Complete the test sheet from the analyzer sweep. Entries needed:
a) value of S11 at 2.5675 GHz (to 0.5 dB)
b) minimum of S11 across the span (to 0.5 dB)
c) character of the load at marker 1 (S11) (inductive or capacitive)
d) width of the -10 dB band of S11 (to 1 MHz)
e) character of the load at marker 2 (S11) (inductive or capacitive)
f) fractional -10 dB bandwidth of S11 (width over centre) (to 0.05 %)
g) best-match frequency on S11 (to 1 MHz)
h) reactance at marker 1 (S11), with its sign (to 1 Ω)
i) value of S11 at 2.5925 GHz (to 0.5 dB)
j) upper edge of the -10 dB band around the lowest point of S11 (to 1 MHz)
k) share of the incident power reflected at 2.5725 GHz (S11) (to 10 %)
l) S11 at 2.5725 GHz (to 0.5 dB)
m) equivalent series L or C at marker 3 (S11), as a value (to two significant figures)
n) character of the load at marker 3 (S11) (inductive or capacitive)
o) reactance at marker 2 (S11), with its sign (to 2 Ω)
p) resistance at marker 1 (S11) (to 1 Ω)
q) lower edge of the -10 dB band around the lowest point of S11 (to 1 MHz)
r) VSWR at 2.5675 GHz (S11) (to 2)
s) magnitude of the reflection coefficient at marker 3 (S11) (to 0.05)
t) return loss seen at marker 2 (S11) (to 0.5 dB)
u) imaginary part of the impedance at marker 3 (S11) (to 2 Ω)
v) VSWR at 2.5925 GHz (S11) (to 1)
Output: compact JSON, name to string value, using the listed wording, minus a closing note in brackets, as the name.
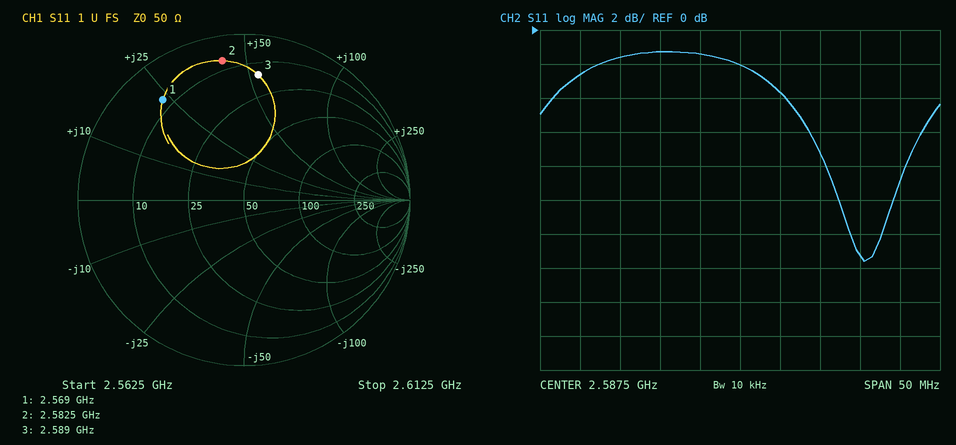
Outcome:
{"value of S11 at 2.5675 GHz": "-2.5 dB", "minimum of S11 across the span": "-13.5 dB", "character of the load at marker 1 (S11)": "inductive", "width of the -10 dB band of S11": "7 MHz", "character of the load at marker 2 (S11)": "inductive", "fractional -10 dB bandwidth of S11 (width over centre)": "0.25 %", "best-match frequency on S11": "2.603 GHz", "reactance at marker 1 (S11), with its sign": "+23 Ω", "value of S11 at 2.5925 GHz": "-3.5 dB", "upper edge of the -10 dB band around the lowest point of S11": "2.607 GHz", "share of the incident power reflected at 2.5725 GHz (S11)": "70 %", "S11 at 2.5725 GHz": "-1.5 dB", "equivalent series L or C at marker 3 (S11), as a value": "3.3 nH", "character of the load at marker 3 (S11)": "inductive", "reactance at marker 2 (S11), with its sign": "+42 Ω", "resistance at marker 1 (S11)": "8 Ω", "lower edge of the -10 dB band around the lowest point of S11": "2.600 GHz", "VSWR at 2.5675 GHz (S11)": "6", "magnitude of the reflection coefficient at marker 3 (S11)": "0.75", "return loss seen at marker 2 (S11)": "1.5 dB", "imaginary part of the impedance at marker 3 (S11)": "+54 Ω", "VSWR at 2.5925 GHz (S11)": "5"}
